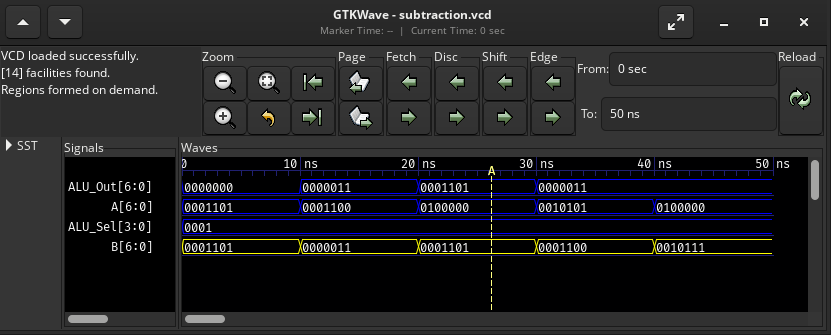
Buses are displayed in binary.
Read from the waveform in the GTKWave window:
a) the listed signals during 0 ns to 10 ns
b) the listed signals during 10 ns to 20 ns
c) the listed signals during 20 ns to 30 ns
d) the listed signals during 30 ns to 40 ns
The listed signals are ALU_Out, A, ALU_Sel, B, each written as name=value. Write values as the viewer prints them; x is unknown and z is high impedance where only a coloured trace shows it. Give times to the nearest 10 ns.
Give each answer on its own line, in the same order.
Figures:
ALU_Out=0000000, A=0001101, ALU_Sel=0001, B=0001101
ALU_Out=0000011, A=0001100, ALU_Sel=0001, B=0000011
ALU_Out=0001101, A=0100000, ALU_Sel=0001, B=0001101
ALU_Out=0000011, A=0010101, ALU_Sel=0001, B=0001100
